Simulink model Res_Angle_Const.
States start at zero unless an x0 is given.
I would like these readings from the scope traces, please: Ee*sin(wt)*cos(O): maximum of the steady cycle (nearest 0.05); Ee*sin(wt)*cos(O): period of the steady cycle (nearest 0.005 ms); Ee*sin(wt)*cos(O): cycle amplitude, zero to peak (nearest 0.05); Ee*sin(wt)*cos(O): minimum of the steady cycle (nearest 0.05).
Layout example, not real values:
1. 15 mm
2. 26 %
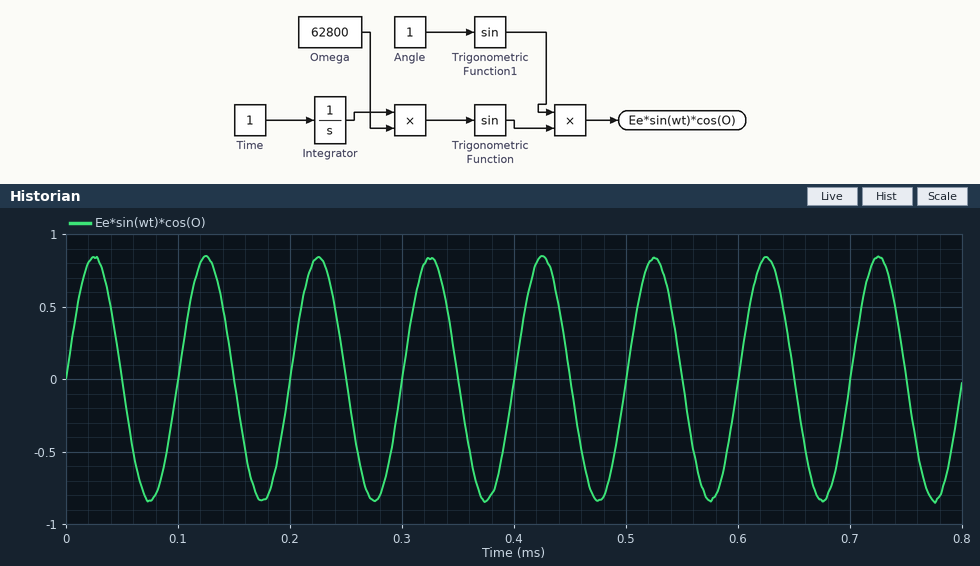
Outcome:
1. 0.85
2. 0.100 ms
3. 0.85
4. -0.85
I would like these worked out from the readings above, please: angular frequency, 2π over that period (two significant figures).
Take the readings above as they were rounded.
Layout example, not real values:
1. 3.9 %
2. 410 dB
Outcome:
1. 63 rad/ms
